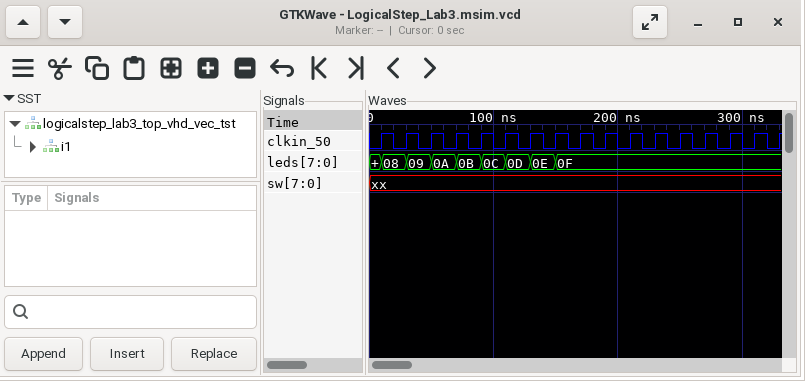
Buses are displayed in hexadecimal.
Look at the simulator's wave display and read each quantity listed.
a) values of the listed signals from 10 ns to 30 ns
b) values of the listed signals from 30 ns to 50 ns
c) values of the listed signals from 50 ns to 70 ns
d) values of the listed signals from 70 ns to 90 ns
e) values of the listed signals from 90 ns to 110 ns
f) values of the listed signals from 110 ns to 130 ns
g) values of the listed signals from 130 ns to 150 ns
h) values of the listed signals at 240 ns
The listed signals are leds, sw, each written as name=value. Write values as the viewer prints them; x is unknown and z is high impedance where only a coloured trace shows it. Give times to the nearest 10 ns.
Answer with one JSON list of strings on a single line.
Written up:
["leds=08, sw=xx", "leds=09, sw=xx", "leds=0A, sw=xx", "leds=0B, sw=xx", "leds=0C, sw=xx", "leds=0D, sw=xx", "leds=0E, sw=xx", "leds=0F, sw=xx"]
